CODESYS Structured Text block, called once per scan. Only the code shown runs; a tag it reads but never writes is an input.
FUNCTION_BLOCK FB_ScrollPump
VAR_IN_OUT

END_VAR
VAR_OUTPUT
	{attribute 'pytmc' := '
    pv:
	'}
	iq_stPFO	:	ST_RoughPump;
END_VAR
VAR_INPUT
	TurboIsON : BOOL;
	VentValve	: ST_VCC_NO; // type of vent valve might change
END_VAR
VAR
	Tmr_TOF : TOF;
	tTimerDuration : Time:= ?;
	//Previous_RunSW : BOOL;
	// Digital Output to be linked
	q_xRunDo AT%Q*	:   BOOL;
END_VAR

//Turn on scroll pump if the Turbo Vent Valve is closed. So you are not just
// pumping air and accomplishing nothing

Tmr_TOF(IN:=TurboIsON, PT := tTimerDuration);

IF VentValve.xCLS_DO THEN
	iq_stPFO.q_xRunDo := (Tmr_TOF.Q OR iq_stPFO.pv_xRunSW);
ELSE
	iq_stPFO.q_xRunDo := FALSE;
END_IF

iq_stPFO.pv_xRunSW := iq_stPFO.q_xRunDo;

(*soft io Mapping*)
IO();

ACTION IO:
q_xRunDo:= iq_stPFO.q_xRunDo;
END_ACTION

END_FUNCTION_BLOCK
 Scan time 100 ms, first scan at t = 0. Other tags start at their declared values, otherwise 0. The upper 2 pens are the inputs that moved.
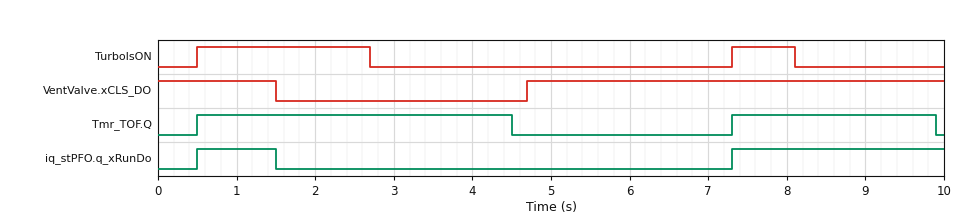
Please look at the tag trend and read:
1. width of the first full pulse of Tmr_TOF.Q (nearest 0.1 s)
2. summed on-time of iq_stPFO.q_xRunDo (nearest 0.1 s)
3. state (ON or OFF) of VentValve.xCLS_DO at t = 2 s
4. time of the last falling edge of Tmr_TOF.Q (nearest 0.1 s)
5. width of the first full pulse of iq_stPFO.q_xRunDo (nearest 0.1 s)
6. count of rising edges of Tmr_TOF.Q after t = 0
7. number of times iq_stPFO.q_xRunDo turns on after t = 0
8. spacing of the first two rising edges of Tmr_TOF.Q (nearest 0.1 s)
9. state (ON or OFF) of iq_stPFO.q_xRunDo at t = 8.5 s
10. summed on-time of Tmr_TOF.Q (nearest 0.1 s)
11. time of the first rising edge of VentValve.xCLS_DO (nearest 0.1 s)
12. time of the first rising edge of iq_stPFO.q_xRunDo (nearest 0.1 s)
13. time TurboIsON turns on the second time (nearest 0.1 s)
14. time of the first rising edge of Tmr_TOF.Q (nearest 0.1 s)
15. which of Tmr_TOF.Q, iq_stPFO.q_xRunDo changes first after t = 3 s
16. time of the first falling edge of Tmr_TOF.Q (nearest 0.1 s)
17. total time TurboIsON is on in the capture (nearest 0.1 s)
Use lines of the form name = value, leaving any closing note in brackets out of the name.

width of the first full pulse of Tmr_TOF.Q = 4.0 s
summed on-time of iq_stPFO.q_xRunDo = 3.7 s
state (ON or OFF) of VentValve.xCLS_DO at t = 2 s = OFF
time of the last falling edge of Tmr_TOF.Q = 9.9 s
width of the first full pulse of iq_stPFO.q_xRunDo = 1.0 s
count of rising edges of Tmr_TOF.Q after t = 0 = 2
number of times iq_stPFO.q_xRunDo turns on after t = 0 = 2
spacing of the first two rising edges of Tmr_TOF.Q = 6.8 s
state (ON or OFF) of iq_stPFO.q_xRunDo at t = 8.5 s = ON
summed on-time of Tmr_TOF.Q = 6.6 s
time of the first rising edge of VentValve.xCLS_DO = 4.7 s
time of the first rising edge of iq_stPFO.q_xRunDo = 0.5 s
time TurboIsON turns on the second time = 7.3 s
time of the first rising edge of Tmr_TOF.Q = 0.5 s
which of Tmr_TOF.Q, iq_stPFO.q_xRunDo changes first after t = 3 s = Tmr_TOF.Q
time of the first falling edge of Tmr_TOF.Q = 4.5 s
total time TurboIsON is on in the capture = 3.0 s
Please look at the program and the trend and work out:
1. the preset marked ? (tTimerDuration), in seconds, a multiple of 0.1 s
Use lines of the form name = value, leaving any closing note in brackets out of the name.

the preset marked ? (tTimerDuration), in seconds, a multiple of 0.1 s = 1.8 s
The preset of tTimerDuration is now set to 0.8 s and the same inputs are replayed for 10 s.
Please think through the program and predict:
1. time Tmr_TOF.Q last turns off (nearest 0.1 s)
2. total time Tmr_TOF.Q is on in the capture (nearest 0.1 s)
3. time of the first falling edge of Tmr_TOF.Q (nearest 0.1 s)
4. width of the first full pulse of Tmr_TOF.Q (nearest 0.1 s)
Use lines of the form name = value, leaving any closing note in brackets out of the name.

time Tmr_TOF.Q last turns off = 8.9 s
total time Tmr_TOF.Q is on in the capture = 4.6 s
time of the first falling edge of Tmr_TOF.Q = 3.5 s
width of the first full pulse of Tmr_TOF.Q = 3.0 s
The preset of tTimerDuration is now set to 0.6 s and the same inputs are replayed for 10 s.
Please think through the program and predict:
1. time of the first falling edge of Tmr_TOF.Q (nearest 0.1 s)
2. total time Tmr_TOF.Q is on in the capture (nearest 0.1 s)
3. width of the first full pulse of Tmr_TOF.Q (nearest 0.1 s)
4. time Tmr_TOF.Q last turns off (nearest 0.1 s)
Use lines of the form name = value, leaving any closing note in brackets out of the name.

time of the first falling edge of Tmr_TOF.Q = 3.3 s
total time Tmr_TOF.Q is on in the capture = 4.2 s
width of the first full pulse of Tmr_TOF.Q = 2.8 s
time Tmr_TOF.Q last turns off = 8.7 s
